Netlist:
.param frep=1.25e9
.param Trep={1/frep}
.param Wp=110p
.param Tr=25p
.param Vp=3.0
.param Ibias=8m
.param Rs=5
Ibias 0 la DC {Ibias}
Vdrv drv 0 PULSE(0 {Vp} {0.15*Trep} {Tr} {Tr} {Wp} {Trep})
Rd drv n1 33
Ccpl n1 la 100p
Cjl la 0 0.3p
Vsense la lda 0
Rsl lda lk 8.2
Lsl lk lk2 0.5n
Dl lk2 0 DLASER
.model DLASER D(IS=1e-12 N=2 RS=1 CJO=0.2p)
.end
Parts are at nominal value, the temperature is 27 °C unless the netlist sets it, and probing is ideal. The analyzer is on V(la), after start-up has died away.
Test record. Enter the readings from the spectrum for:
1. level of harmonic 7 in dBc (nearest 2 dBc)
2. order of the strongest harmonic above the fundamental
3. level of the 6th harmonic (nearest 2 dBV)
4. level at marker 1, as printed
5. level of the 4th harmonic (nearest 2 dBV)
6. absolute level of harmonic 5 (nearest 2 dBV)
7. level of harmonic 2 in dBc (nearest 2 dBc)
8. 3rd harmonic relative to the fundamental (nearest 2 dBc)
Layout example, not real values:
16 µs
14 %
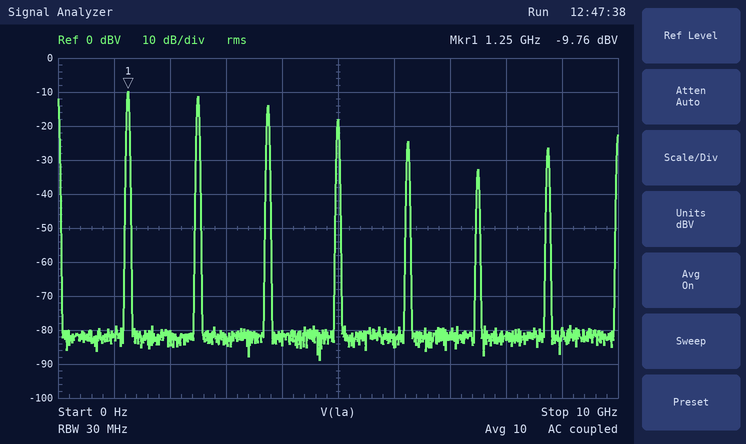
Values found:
-16 dBc
2
-32 dBV
-9.76 dBV
-18 dBV
-24 dBV
-2 dBc
-4 dBc
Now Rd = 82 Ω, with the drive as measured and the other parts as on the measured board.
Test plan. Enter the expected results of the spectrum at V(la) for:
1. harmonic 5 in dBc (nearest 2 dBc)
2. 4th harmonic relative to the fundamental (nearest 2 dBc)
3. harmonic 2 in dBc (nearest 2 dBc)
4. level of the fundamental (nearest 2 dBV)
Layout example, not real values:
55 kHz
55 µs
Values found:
-10 dBc
-4 dBc
0 dBc
-20 dBV
